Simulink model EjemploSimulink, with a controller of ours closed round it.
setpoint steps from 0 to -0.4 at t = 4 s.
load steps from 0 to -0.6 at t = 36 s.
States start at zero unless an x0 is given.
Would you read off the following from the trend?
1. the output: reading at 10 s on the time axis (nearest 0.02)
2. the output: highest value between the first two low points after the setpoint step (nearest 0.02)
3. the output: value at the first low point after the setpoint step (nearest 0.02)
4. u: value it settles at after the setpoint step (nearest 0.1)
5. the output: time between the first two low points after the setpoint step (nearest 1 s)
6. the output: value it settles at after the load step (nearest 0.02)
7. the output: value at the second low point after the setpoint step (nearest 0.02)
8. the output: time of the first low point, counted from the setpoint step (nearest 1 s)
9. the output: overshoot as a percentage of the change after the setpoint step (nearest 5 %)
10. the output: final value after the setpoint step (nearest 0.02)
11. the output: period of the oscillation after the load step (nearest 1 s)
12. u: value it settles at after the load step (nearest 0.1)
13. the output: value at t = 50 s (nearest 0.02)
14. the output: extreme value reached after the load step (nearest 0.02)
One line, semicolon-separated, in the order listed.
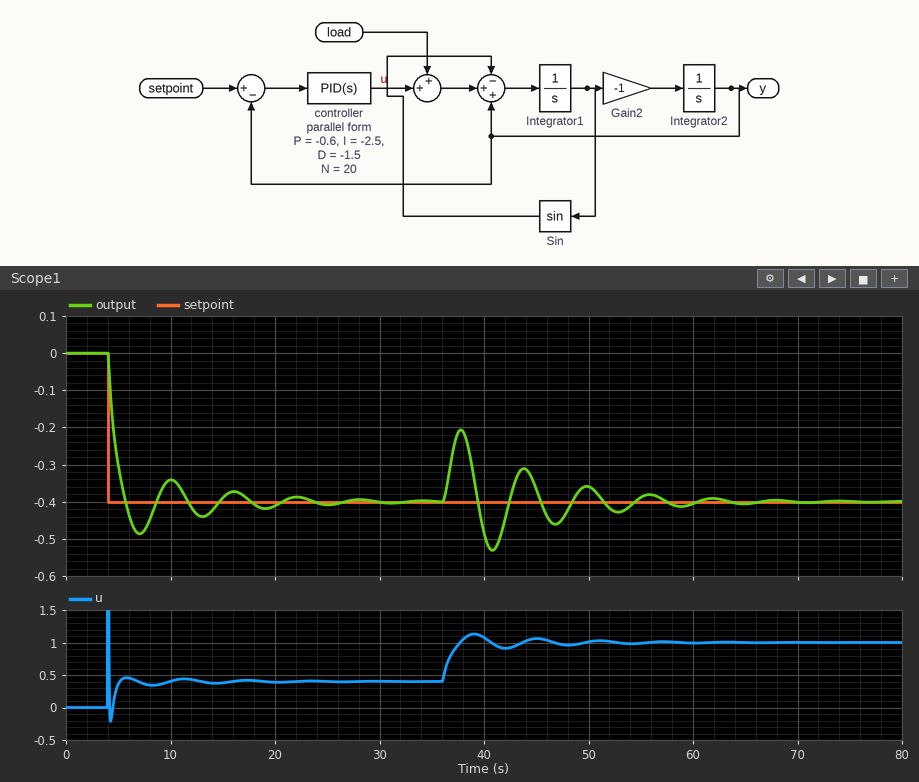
-0.34; -0.34; -0.48; 0.4; 6 s; -0.40; -0.44; 3 s; 20 %; -0.40; 6 s; 1.0; -0.36; -0.20
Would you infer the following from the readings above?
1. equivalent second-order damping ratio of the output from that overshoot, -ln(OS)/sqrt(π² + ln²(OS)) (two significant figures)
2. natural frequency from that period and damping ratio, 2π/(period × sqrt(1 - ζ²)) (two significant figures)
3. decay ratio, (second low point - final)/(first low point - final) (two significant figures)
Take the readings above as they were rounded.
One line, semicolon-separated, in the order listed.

0.46; 1.2 rad/s; 0.50
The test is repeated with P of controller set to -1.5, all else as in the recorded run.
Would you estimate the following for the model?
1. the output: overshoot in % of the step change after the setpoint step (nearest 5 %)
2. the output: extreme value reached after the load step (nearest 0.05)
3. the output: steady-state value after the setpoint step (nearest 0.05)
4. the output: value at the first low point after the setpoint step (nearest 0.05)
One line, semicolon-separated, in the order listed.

10 %; -0.25; -0.40; -0.45
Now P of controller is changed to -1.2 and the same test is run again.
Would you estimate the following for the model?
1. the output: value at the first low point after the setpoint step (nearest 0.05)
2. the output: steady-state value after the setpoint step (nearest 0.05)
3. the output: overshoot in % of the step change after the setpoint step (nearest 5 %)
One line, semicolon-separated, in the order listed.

-0.45; -0.40; 15 %
